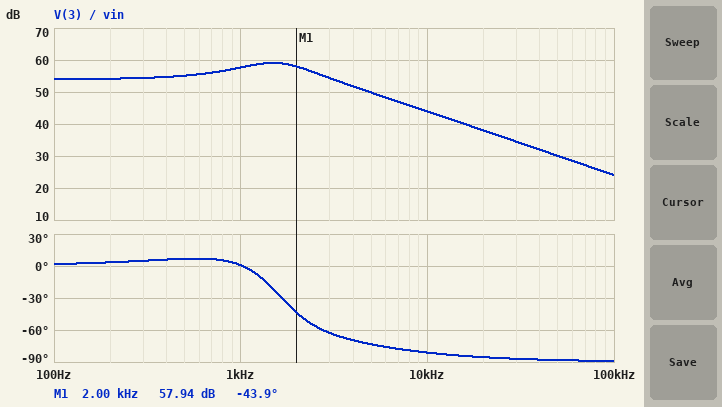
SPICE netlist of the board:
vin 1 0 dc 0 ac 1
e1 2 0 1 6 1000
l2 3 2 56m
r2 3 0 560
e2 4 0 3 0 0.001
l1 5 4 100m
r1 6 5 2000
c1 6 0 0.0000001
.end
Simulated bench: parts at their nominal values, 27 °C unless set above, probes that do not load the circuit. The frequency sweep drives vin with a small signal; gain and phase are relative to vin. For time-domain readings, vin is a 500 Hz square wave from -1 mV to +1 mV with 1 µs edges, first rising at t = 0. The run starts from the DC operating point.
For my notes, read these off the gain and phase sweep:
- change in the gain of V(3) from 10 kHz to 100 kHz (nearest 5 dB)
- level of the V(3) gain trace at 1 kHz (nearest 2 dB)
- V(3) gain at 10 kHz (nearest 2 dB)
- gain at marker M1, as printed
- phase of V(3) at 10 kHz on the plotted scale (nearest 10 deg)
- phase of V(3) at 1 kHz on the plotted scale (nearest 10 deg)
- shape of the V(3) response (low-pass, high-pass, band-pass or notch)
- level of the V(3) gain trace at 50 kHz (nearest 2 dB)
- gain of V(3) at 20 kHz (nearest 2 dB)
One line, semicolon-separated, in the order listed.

-20 dB; 58 dB; 44 dB; 57.94 dB; -80 deg; 0 deg; low-pass; 30 dB; 38 dB
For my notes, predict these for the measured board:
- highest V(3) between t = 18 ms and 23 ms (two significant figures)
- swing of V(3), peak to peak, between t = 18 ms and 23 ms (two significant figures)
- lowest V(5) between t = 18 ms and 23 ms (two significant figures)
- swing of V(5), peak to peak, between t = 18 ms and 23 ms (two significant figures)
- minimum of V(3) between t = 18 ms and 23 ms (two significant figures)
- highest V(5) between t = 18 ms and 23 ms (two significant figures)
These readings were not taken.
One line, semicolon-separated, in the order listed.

960 mV; 1.9 V; -1.1 mV; 2.2 mV; -960 mV; 1.1 mV
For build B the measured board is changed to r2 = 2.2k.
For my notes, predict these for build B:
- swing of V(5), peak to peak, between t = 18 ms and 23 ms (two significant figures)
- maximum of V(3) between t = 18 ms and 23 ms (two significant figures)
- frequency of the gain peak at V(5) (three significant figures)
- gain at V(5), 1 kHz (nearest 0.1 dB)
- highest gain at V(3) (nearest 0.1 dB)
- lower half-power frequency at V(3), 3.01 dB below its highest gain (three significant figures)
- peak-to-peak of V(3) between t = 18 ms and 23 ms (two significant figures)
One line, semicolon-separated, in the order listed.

2.6 mV; 1.3 V; 1.99 kHz; -1.7 dB; 61.0 dB; 1.19 kHz; 2.6 V
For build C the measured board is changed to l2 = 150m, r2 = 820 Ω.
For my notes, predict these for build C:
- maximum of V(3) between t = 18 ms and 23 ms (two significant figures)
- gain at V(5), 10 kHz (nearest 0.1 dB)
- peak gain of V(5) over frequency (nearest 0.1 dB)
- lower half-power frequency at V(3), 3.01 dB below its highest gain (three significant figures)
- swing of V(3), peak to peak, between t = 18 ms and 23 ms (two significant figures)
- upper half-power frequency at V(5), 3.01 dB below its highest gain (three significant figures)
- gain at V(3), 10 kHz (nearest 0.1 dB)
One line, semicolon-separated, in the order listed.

780 mV; -31.4 dB; -1.6 dB; 169 Hz; 1.6 V; 1.77 kHz; 38.8 dB
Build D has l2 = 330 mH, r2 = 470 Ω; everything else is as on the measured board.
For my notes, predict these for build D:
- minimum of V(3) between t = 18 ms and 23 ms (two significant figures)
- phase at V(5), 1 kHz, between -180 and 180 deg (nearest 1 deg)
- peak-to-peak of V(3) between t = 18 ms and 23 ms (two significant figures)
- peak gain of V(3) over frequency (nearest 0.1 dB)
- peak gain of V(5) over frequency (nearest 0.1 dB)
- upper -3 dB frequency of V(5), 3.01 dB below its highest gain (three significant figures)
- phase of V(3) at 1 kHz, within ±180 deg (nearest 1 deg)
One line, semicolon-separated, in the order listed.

-500 mV; -84 deg; 1.0 V; 54.0 dB; -6.0 dB; 786 Hz; -71 deg
